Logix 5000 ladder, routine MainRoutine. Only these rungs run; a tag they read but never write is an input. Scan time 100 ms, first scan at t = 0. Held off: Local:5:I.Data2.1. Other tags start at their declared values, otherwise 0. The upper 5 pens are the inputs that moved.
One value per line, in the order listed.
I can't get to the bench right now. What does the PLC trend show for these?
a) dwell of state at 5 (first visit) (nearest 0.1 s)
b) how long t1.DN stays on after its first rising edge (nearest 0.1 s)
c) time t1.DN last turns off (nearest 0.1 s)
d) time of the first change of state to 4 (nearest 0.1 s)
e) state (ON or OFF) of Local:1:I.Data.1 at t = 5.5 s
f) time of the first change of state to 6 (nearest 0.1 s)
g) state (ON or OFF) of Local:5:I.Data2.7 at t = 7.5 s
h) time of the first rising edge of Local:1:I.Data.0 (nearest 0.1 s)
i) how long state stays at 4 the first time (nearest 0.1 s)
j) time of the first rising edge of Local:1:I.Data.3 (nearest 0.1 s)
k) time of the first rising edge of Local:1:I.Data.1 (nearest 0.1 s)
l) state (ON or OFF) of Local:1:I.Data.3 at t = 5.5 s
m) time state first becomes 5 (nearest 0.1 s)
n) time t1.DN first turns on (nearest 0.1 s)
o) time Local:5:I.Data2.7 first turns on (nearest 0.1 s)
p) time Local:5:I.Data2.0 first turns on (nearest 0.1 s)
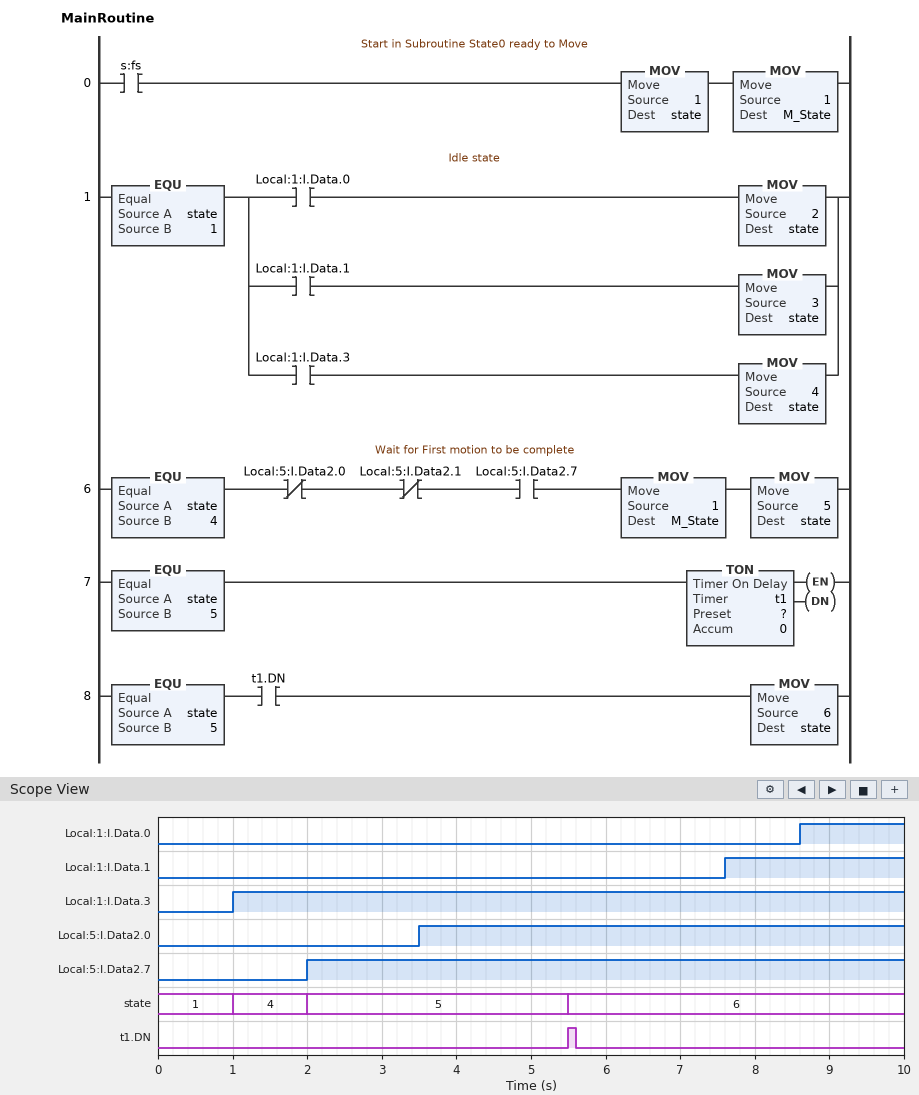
3.5 s
0.1 s
5.6 s
1.0 s
OFF
5.5 s
ON
8.6 s
1.0 s
1.0 s
7.6 s
ON
2.0 s
5.5 s
2.0 s
3.5 s
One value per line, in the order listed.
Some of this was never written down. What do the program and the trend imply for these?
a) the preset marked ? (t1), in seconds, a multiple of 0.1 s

3.5 s
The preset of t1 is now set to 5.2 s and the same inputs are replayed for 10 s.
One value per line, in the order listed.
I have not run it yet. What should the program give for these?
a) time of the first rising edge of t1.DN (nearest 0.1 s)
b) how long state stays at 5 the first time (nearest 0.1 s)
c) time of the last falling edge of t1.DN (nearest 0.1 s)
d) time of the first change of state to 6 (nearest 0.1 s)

7.2 s
5.2 s
7.3 s
7.2 s
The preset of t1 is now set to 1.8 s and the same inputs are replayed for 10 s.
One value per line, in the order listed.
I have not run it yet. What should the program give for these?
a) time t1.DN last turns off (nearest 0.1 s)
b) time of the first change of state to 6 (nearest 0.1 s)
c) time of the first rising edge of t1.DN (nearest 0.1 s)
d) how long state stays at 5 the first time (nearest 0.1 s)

3.9 s
3.8 s
3.8 s
1.8 s
